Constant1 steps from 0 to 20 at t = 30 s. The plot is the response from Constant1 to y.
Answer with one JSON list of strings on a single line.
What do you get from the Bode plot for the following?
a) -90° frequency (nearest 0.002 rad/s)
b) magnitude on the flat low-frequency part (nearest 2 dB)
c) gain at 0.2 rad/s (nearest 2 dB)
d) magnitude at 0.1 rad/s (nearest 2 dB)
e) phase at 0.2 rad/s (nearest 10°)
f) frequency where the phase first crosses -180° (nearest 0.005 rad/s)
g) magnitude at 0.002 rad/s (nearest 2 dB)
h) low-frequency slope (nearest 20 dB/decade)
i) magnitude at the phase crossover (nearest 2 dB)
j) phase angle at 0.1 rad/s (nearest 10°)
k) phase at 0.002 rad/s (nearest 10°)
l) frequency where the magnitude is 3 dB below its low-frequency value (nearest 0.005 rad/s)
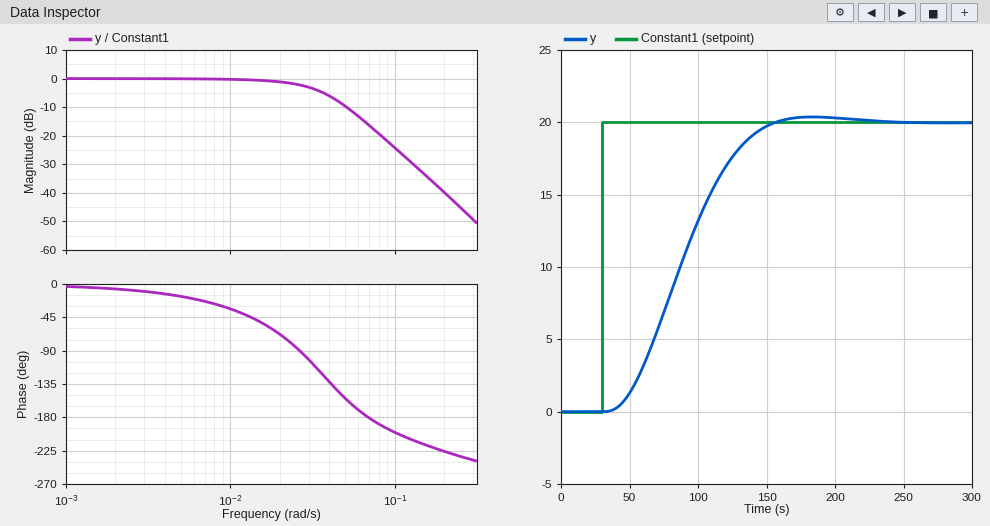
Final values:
["0.026 rad/s", "0 dB", "-40 dB", "-24 dB", "-230°", "0.070 rad/s", "0 dB", "0 dB/decade", "-16 dB", "-200°", "-10°", "0.030 rad/s"]
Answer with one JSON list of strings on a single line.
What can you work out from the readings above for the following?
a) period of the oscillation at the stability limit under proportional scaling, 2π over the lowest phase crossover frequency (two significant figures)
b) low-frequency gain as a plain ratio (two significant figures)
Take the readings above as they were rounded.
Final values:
["90 s", "1.0"]
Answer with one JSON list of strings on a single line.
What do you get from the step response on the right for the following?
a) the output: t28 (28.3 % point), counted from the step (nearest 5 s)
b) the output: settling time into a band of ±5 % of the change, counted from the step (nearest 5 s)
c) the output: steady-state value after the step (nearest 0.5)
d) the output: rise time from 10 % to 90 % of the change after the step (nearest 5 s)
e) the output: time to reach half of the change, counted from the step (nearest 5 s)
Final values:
["40 s", "110 s", "20.0", "75 s", "55 s"]
